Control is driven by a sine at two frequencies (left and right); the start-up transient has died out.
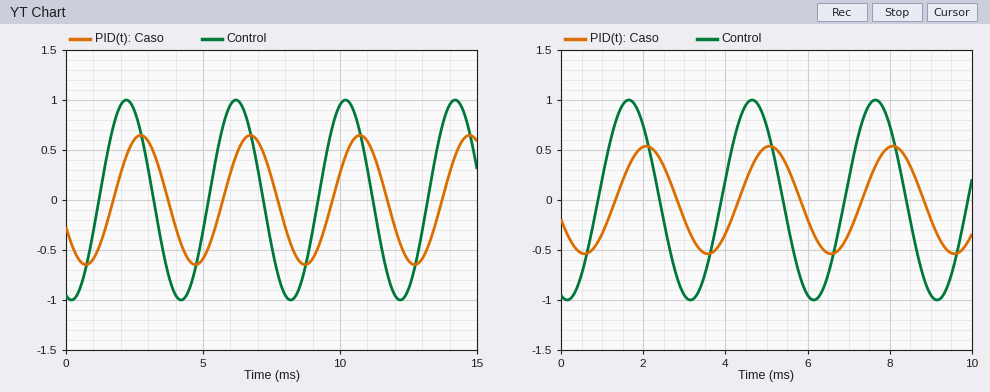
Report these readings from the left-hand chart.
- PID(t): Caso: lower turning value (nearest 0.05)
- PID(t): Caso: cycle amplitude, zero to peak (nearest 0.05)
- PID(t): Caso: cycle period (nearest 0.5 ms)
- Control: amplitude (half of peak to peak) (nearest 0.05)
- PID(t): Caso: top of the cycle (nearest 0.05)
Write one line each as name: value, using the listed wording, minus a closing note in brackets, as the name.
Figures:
PID(t): Caso: lower turning value: -0.65
PID(t): Caso: cycle amplitude, zero to peak: 0.65
PID(t): Caso: cycle period: 4.0 ms
Control: amplitude (half of peak to peak): 1.00
PID(t): Caso: top of the cycle: 0.65
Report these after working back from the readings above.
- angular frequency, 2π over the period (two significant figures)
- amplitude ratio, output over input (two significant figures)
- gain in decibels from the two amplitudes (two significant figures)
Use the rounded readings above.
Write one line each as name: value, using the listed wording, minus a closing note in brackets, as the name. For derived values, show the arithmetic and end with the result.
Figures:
angular frequency, 2π over the period: 2π / 4 = 1.6 rad/ms
amplitude ratio, output over input: 0.65 / 1 = 0.65
gain in decibels from the two amplitudes: 20 log10(0.65 / 1) = -3.7 dB
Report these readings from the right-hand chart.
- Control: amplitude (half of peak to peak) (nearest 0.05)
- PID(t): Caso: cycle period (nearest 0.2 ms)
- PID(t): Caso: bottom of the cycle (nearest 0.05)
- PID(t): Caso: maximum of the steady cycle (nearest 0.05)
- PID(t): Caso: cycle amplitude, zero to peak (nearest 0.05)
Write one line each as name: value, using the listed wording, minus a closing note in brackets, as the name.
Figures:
Control: amplitude (half of peak to peak): 1.00
PID(t): Caso: cycle period: 3.0 ms
PID(t): Caso: bottom of the cycle: -0.55
PID(t): Caso: maximum of the steady cycle: 0.55
PID(t): Caso: cycle amplitude, zero to peak: 0.55
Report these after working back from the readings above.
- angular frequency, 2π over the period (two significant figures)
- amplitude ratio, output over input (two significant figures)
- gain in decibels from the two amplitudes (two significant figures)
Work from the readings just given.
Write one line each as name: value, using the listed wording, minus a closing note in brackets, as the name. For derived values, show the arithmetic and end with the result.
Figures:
angular frequency, 2π over the period: 2π / 3 = 2.1 rad/ms
amplitude ratio, output over input: 0.55 / 1 = 0.55
gain in decibels from the two amplitudes: 20 log10(0.55 / 1) = -5.2 dB
